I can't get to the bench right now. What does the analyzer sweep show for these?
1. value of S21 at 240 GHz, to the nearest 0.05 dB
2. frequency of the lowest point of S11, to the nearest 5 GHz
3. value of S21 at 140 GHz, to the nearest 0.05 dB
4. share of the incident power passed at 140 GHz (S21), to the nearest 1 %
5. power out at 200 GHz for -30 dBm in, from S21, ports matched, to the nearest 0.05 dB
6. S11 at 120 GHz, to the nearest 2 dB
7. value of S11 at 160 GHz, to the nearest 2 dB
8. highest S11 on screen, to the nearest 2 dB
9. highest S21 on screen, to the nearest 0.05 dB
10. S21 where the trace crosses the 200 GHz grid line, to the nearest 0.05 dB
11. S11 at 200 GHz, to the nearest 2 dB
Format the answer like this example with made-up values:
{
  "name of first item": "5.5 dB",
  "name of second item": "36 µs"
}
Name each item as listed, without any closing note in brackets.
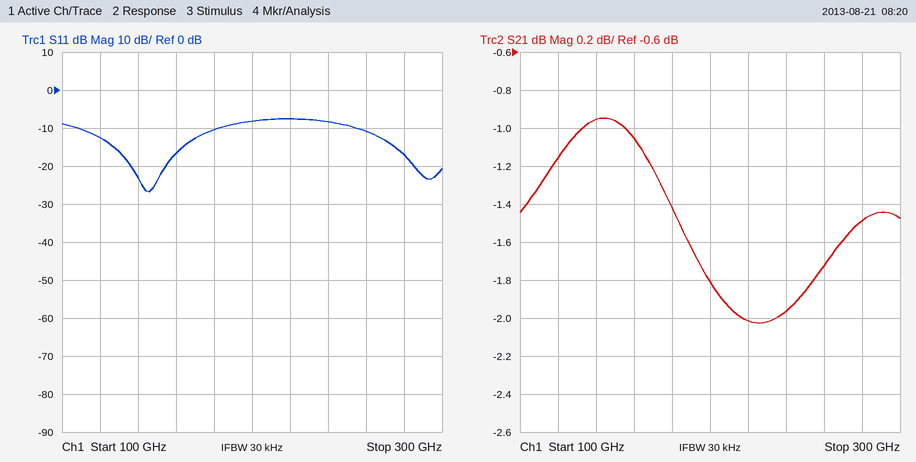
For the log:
{
  "value of S21 at 240 GHz, to the nearest 0.05 dB": "-1.95 dB",
  "frequency of the lowest point of S11, to the nearest 5 GHz": "145 GHz",
  "value of S21 at 140 GHz, to the nearest 0.05 dB": "-0.95 dB",
  "share of the incident power passed at 140 GHz (S21), to the nearest 1 %": "80 %",
  "power out at 200 GHz for -30 dBm in, from S21, ports matched, to the nearest 0.05 dB": "-31.80 dBm",
  "S11 at 120 GHz, to the nearest 2 dB": "-12 dB",
  "value of S11 at 160 GHz, to the nearest 2 dB": "-16 dB",
  "highest S11 on screen, to the nearest 2 dB": "-8 dB",
  "highest S21 on screen, to the nearest 0.05 dB": "-0.95 dB",
  "S21 where the trace crosses the 200 GHz grid line, to the nearest 0.05 dB": "-1.80 dB",
  "S11 at 200 GHz, to the nearest 2 dB": "-8 dB"
}
